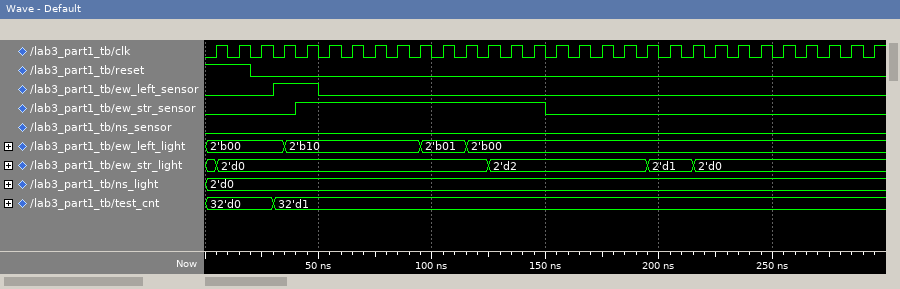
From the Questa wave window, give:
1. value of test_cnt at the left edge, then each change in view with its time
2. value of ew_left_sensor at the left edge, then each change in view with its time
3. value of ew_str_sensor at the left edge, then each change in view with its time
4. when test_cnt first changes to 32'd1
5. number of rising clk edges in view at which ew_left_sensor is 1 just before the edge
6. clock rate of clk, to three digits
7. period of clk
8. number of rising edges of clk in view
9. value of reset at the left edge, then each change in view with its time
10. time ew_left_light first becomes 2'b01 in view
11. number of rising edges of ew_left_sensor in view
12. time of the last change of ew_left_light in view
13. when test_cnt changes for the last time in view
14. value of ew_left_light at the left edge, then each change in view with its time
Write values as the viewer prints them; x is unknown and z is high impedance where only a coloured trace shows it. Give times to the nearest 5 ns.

32'd0, 32'd1 at 30 ns
0, 1 at 30 ns, 0 at 50 ns
0, 1 at 40 ns, 0 at 150 ns
30 ns
2
100 MHz
10 ns
30
1, 0 at 20 ns
95 ns
1
115 ns
30 ns
2'b00, 2'b10 at 35 ns, 2'b01 at 95 ns, 2'b00 at 115 ns
